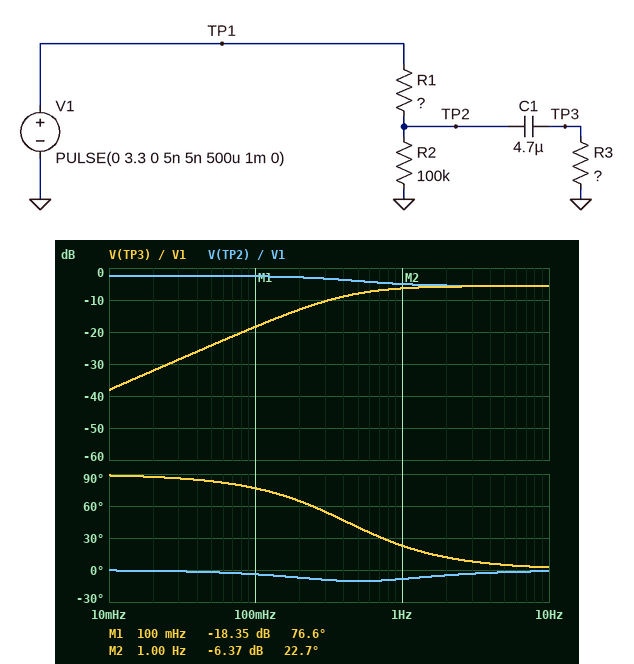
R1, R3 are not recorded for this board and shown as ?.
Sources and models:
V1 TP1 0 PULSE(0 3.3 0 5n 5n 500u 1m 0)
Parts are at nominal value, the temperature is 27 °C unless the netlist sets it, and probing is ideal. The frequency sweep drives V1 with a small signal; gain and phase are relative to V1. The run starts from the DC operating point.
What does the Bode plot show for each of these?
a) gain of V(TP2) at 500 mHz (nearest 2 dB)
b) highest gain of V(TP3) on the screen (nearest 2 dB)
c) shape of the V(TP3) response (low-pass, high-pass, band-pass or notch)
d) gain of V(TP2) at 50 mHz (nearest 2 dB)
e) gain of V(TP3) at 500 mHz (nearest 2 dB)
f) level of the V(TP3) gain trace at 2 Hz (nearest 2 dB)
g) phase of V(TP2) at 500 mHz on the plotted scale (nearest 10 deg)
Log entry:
-4 dB
-6 dB
high-pass
-2 dB
-8 dB
-6 dB
-10 deg
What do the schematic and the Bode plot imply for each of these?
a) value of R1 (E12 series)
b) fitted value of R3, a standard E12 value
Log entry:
33 kΩ
56 kΩ
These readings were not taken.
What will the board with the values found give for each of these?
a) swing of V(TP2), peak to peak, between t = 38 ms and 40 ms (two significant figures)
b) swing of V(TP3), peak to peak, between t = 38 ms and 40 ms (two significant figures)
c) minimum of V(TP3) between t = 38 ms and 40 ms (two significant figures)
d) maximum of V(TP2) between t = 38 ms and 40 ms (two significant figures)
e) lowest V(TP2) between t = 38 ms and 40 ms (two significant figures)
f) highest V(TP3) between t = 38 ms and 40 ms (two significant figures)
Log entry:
1.7 V
1.7 V
-86 mV
1.8 V
36 mV
1.6 V
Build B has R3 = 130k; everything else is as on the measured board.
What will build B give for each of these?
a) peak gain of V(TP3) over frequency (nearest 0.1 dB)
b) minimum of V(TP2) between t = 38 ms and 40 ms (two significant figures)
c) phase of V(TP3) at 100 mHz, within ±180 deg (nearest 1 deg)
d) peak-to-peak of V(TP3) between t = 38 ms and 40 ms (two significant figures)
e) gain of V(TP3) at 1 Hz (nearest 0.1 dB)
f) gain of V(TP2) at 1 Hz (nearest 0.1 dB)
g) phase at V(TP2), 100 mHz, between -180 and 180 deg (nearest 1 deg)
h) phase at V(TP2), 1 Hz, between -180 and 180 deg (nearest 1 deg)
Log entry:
-4.0 dB
10 mV
65 deg
2.1 V
-4.2 dB
-3.9 dB
-4 deg
-2 deg
